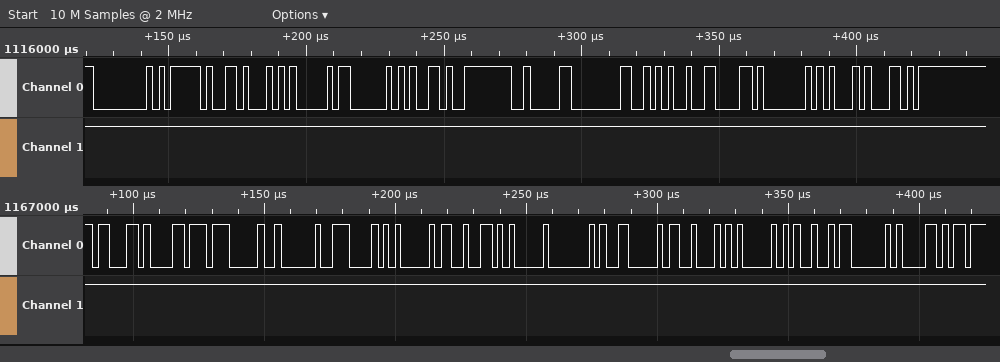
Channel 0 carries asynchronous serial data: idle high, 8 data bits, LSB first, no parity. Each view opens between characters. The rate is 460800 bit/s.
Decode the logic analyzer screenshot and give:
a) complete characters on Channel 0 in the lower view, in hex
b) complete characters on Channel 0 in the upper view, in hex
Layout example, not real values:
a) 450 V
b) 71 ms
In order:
a) 63, D8, 07, 02, 0E, 05, 93, 05, 40, 06, 13, 05, 25, 03, 61
b) 00, 7D, 16, 05, 03, 65, FE, 82, 80, 2A, 86, 01, 45, AC
